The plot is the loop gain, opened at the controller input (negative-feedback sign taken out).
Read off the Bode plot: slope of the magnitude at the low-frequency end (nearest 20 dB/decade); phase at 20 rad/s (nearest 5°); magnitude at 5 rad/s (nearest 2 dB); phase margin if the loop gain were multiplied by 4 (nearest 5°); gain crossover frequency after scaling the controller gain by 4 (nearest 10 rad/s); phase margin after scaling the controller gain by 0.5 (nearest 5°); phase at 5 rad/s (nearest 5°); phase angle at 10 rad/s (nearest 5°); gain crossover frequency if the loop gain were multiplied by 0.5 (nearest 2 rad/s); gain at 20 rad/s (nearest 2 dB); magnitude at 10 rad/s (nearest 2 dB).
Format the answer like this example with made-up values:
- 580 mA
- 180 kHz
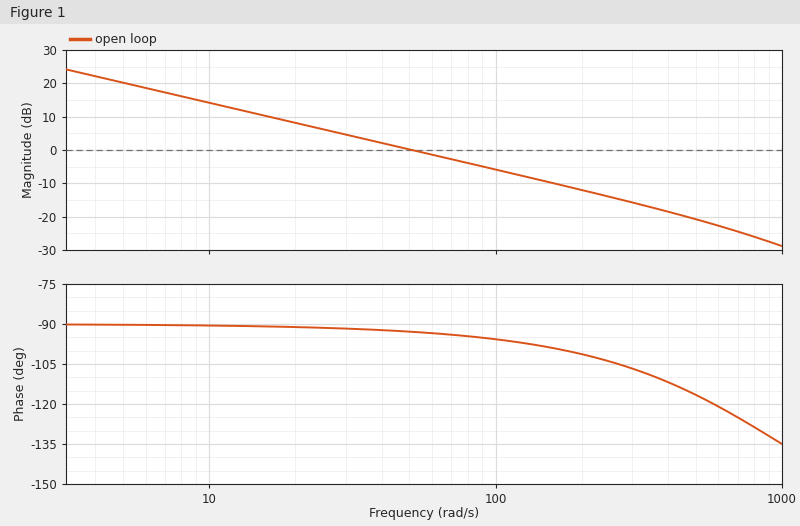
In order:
- -20 dB/decade
- -90°
- 20 dB
- 80°
- 200 rad/s
- 90°
- -90°
- -90°
- 26 rad/s
- 8 dB
- 14 dB
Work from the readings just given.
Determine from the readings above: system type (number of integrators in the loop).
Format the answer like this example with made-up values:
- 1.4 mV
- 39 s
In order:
- 1
